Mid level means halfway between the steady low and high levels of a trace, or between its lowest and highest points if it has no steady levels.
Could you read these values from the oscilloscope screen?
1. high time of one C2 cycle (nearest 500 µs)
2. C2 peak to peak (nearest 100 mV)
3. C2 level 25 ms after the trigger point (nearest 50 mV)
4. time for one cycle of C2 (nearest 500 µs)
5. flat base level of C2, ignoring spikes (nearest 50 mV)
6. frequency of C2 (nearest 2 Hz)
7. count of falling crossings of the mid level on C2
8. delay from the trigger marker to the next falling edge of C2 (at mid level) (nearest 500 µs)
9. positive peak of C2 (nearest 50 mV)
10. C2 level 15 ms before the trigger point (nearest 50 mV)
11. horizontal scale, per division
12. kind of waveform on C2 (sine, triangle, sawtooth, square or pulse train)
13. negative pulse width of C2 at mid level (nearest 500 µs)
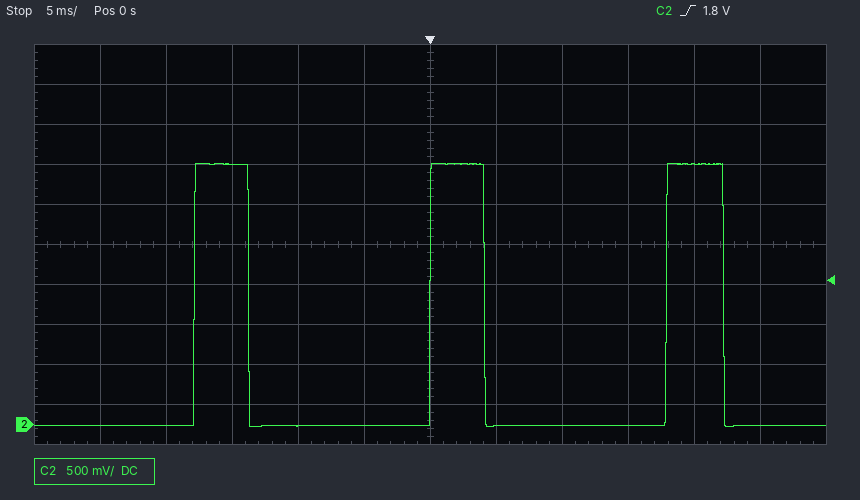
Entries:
4.0 ms
3.30 V
0 mV
18.0 ms
0 mV
56 Hz
3
4.0 ms
3.25 V
3.25 V
5 ms
pulse train
13.5 ms
